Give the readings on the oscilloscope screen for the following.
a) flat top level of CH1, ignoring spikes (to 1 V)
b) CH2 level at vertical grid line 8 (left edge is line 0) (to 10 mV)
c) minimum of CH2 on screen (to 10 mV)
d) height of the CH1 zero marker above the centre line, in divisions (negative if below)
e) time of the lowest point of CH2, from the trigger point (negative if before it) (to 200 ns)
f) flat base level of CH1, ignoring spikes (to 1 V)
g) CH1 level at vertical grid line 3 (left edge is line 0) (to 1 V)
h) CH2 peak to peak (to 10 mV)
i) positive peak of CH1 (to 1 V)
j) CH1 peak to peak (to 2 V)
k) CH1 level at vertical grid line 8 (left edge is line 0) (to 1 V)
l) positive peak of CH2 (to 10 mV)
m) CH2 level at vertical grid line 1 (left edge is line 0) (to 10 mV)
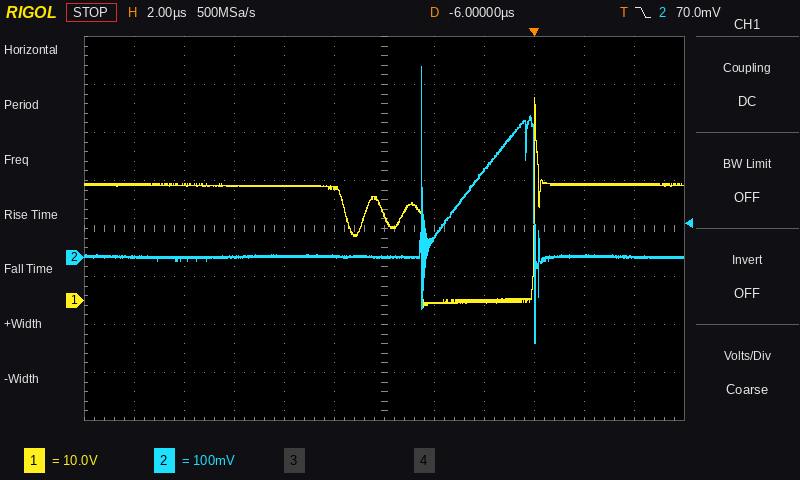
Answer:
24 V
180 mV
-180 mV
-1.5 div
0.0 µs
0 V
24 V
580 mV
42 V
44 V
0 V
400 mV
0 mV
